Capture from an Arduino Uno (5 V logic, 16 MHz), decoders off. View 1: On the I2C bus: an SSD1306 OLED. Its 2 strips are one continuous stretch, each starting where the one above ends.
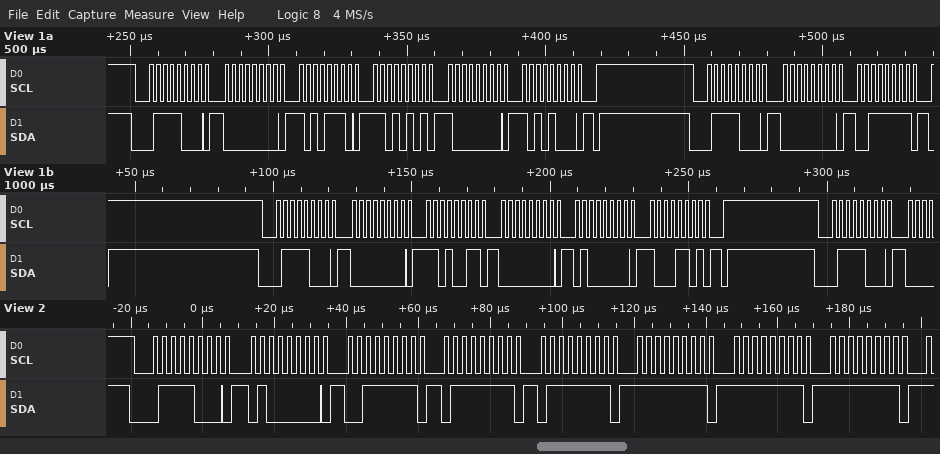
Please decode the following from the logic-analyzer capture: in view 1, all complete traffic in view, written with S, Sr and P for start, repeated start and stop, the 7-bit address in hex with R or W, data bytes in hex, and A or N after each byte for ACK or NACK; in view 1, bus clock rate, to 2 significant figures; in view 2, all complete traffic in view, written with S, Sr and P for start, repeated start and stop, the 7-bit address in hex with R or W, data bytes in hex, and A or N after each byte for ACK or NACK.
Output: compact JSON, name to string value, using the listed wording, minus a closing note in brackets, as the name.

{"in view 1, all complete traffic in view, written with S, Sr and P for start, repeated start and stop, the 7-bit address in hex with R or W, data bytes in hex, and A or N after each byte for ACK or NACK": "S 3CW A 00 A AE A D5 A 80 A A8 A P S 3CW A 00 A 3F A P S 3CW A 00 A D3 A 00 A 40 A 8D A P S 3CW A", "in view 1, bus clock rate, to 2 significant figures": "400 kHz", "in view 2, all complete traffic in view, written with S, Sr and P for start, repeated start and stop, the 7-bit address in hex with R or W, data bytes in hex, and A or N after each byte for ACK or NACK": "S 3CW A 40 A 3F A 7F A 7F A FF A FF A FF A"}
